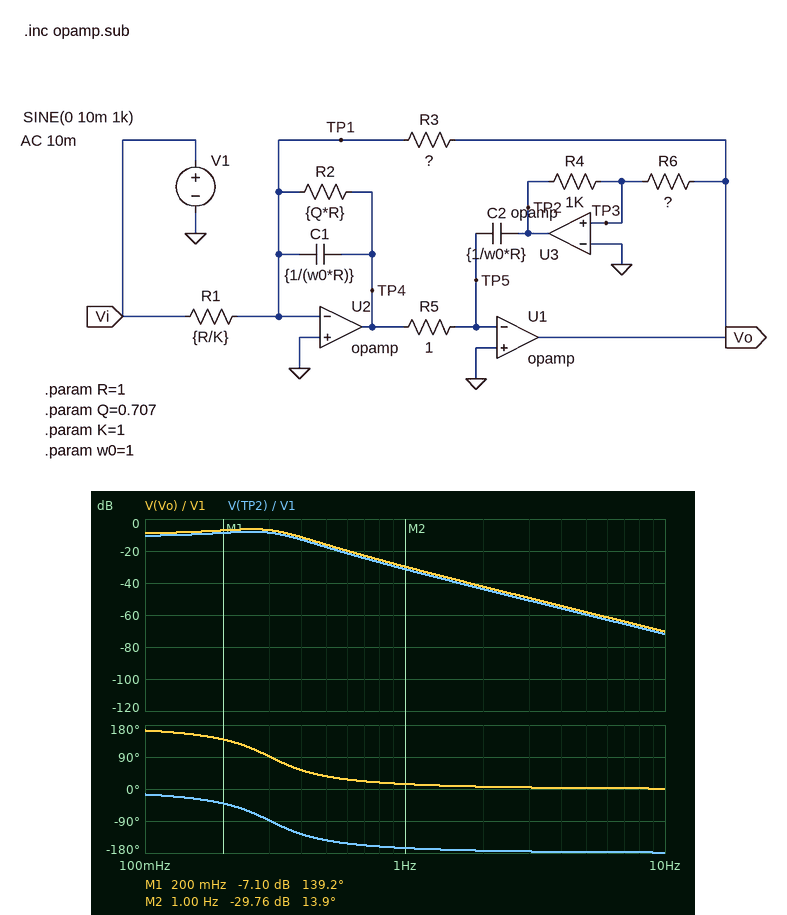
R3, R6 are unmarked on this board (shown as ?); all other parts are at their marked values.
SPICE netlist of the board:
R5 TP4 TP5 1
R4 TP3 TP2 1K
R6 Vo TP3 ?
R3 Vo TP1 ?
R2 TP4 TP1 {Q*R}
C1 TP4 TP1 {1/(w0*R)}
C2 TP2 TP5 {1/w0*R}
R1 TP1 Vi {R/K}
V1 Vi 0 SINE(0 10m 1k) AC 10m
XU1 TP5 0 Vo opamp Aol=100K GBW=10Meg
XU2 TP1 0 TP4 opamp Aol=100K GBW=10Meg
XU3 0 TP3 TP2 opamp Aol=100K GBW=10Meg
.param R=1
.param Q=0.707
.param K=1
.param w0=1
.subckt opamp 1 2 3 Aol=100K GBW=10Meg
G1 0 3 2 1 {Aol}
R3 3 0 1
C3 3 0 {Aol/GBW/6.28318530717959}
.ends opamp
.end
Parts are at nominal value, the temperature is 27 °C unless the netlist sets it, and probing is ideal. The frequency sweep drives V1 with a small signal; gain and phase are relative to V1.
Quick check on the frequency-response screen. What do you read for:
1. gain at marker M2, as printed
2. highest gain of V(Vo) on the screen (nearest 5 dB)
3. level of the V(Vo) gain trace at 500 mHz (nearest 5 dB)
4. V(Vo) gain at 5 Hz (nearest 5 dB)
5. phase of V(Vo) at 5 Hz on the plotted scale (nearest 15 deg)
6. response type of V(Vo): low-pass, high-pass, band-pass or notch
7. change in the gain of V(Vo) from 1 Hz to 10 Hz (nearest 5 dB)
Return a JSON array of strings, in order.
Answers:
["-29.76 dB", "-5 dB", "-15 dB", "-60 dB", "0 deg", "low-pass", "-40 dB"]
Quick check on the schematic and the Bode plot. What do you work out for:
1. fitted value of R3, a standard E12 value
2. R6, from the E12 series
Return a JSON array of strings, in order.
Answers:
["0.33 Ω", "1.2 kΩ"]
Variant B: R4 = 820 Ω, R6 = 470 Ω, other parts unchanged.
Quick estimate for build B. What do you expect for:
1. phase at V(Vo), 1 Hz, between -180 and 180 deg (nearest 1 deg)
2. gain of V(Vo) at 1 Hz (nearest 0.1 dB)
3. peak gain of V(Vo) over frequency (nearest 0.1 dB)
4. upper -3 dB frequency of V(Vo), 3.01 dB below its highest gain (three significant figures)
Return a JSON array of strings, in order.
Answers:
["13 deg", "-36.6 dB", "-8.8 dB", "242 mHz"]
